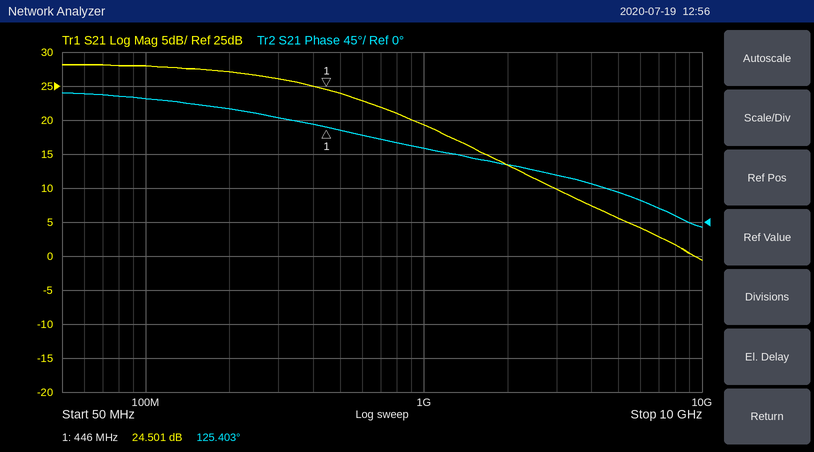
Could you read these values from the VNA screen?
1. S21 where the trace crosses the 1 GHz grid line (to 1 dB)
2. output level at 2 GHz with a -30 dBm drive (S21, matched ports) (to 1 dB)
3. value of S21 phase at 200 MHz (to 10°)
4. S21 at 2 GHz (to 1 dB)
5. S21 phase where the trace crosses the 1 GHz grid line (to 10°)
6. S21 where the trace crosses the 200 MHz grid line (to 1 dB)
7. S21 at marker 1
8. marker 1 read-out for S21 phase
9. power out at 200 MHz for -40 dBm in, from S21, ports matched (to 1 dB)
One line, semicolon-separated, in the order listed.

19 dB; -17 dBm; 150°; 13 dB; 100°; 27 dB; 24.501 dB; 125.403°; -13 dBm
